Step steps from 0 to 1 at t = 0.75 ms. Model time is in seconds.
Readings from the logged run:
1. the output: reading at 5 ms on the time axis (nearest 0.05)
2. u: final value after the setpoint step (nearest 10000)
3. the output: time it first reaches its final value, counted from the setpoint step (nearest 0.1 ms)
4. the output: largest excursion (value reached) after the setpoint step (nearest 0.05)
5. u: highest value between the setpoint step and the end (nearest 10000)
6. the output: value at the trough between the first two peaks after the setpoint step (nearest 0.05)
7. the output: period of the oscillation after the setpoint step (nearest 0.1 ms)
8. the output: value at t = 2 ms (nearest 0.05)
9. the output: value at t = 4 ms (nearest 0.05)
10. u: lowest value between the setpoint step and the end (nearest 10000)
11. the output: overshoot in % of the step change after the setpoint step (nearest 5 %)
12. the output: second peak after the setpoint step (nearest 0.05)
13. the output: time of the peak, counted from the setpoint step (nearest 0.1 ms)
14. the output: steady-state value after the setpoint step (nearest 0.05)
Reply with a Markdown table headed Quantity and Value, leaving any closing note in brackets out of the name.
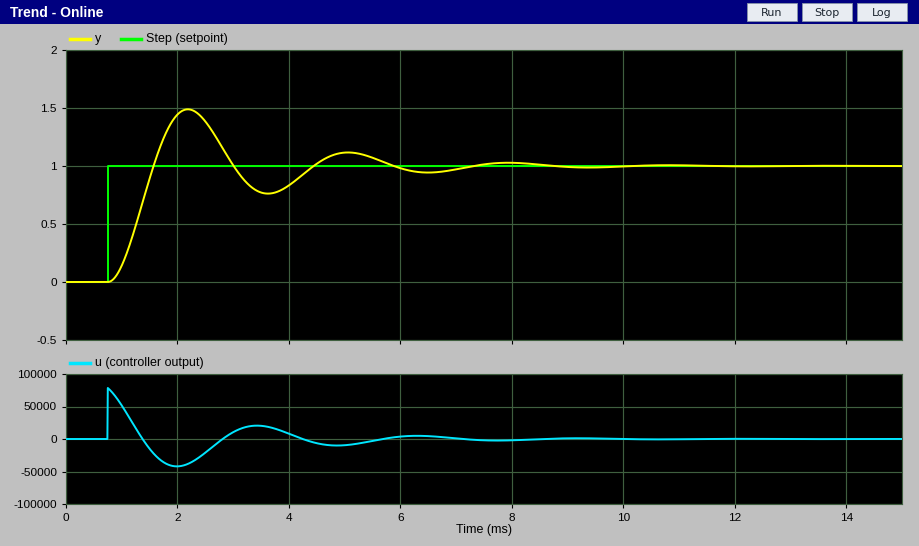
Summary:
| Quantity | Value |
|---|---|
| the output: reading at 5 ms on the time axis | 1.10 |
| u: final value after the setpoint step | 0 |
| the output: time it first reaches its final value, counted from the setpoint step | 0.8 ms |
| the output: largest excursion (value reached) after the setpoint step | 1.50 |
| u: highest value between the setpoint step and the end | 80000 |
| the output: value at the trough between the first two peaks after the setpoint step | 0.75 |
| the output: period of the oscillation after the setpoint step | 2.9 ms |
| the output: value at t = 2 ms | 1.45 |
| the output: value at t = 4 ms | 0.85 |
| u: lowest value between the setpoint step and the end | -40000 |
| the output: overshoot in % of the step change after the setpoint step | 50 % |
| the output: second peak after the setpoint step | 1.10 |
| the output: time of the peak, counted from the setpoint step | 1.4 ms |
| the output: steady-state value after the setpoint step | 1.00 |
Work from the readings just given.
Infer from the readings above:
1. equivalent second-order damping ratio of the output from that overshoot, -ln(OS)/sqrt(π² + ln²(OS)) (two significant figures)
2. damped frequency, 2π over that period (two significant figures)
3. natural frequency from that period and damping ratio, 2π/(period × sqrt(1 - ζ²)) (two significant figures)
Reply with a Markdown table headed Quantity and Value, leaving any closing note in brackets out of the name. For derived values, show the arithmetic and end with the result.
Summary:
| Quantity | Value |
|---|---|
| equivalent second-order damping ratio of the output from that overshoot, -ln(OS)/sqrt(π² + ln²(OS)) | ln(0.5) = -0.693; 0.693 / sqrt(9.870 + 0.480) = 0.22 |
| damped frequency, 2π over that period | 2π / 2.9 = 2.2 rad/ms |
| natural frequency from that period and damping ratio, 2π/(period × sqrt(1 - ζ²)) | 2π / (2.9 × sqrt(1 - 0.22²)) = 2.2 rad/ms |
